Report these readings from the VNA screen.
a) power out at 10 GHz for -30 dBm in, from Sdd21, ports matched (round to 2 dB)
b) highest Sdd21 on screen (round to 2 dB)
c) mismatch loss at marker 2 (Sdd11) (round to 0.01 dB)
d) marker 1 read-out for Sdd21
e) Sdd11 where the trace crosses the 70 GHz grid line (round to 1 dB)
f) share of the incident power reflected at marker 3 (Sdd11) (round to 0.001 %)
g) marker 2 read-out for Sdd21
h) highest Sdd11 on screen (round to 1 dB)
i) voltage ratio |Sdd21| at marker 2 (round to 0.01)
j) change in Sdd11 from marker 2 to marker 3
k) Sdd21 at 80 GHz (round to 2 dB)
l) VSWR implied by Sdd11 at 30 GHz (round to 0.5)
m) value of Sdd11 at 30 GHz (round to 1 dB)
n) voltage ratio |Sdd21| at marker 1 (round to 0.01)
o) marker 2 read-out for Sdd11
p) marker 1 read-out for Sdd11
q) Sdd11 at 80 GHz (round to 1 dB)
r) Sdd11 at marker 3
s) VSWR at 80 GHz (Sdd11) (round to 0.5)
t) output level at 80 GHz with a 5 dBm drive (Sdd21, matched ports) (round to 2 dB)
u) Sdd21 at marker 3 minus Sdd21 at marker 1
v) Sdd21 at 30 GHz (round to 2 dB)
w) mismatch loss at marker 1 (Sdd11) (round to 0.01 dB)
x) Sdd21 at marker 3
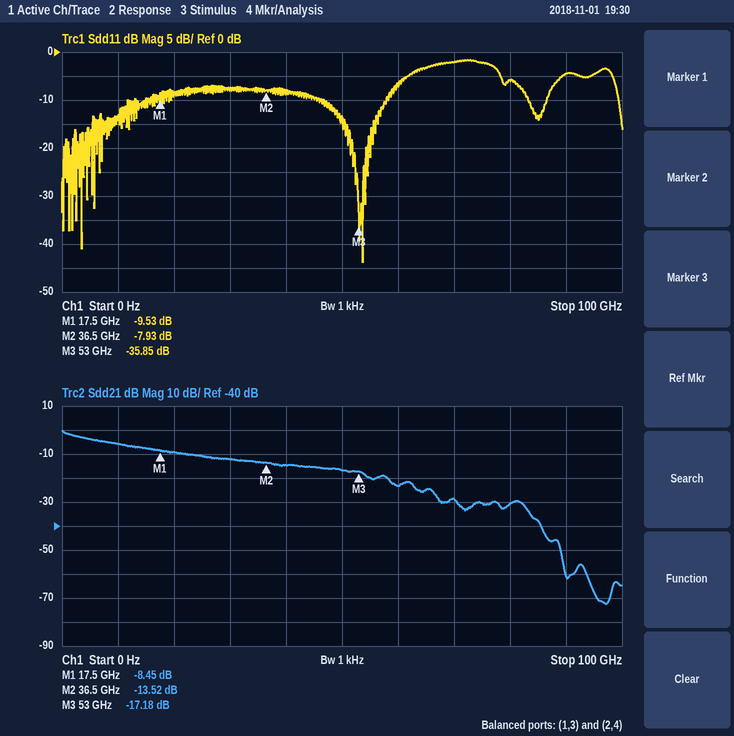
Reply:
-36 dBm
0 dB
0.76 dB
-8.45 dB
-2 dB
0.026 %
-13.52 dB
-2 dB
0.21
-27.92 dB
-30 dB
2.5
-8 dB
0.38
-7.93 dB
-9.53 dB
-6 dB
-35.85 dB
3.0
-26 dBm
-8.73 dB
-12 dB
0.51 dB
-17.18 dB
